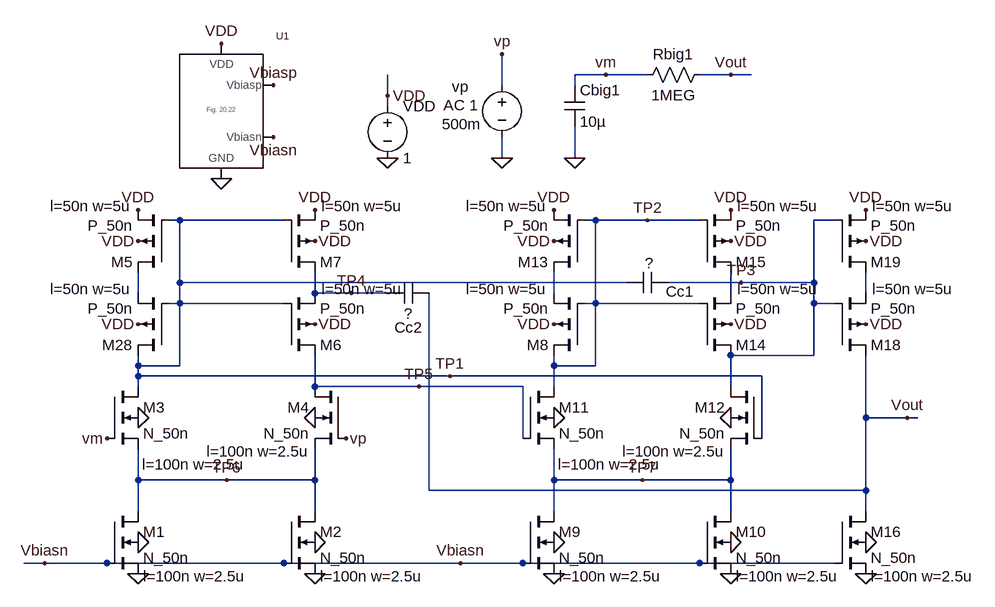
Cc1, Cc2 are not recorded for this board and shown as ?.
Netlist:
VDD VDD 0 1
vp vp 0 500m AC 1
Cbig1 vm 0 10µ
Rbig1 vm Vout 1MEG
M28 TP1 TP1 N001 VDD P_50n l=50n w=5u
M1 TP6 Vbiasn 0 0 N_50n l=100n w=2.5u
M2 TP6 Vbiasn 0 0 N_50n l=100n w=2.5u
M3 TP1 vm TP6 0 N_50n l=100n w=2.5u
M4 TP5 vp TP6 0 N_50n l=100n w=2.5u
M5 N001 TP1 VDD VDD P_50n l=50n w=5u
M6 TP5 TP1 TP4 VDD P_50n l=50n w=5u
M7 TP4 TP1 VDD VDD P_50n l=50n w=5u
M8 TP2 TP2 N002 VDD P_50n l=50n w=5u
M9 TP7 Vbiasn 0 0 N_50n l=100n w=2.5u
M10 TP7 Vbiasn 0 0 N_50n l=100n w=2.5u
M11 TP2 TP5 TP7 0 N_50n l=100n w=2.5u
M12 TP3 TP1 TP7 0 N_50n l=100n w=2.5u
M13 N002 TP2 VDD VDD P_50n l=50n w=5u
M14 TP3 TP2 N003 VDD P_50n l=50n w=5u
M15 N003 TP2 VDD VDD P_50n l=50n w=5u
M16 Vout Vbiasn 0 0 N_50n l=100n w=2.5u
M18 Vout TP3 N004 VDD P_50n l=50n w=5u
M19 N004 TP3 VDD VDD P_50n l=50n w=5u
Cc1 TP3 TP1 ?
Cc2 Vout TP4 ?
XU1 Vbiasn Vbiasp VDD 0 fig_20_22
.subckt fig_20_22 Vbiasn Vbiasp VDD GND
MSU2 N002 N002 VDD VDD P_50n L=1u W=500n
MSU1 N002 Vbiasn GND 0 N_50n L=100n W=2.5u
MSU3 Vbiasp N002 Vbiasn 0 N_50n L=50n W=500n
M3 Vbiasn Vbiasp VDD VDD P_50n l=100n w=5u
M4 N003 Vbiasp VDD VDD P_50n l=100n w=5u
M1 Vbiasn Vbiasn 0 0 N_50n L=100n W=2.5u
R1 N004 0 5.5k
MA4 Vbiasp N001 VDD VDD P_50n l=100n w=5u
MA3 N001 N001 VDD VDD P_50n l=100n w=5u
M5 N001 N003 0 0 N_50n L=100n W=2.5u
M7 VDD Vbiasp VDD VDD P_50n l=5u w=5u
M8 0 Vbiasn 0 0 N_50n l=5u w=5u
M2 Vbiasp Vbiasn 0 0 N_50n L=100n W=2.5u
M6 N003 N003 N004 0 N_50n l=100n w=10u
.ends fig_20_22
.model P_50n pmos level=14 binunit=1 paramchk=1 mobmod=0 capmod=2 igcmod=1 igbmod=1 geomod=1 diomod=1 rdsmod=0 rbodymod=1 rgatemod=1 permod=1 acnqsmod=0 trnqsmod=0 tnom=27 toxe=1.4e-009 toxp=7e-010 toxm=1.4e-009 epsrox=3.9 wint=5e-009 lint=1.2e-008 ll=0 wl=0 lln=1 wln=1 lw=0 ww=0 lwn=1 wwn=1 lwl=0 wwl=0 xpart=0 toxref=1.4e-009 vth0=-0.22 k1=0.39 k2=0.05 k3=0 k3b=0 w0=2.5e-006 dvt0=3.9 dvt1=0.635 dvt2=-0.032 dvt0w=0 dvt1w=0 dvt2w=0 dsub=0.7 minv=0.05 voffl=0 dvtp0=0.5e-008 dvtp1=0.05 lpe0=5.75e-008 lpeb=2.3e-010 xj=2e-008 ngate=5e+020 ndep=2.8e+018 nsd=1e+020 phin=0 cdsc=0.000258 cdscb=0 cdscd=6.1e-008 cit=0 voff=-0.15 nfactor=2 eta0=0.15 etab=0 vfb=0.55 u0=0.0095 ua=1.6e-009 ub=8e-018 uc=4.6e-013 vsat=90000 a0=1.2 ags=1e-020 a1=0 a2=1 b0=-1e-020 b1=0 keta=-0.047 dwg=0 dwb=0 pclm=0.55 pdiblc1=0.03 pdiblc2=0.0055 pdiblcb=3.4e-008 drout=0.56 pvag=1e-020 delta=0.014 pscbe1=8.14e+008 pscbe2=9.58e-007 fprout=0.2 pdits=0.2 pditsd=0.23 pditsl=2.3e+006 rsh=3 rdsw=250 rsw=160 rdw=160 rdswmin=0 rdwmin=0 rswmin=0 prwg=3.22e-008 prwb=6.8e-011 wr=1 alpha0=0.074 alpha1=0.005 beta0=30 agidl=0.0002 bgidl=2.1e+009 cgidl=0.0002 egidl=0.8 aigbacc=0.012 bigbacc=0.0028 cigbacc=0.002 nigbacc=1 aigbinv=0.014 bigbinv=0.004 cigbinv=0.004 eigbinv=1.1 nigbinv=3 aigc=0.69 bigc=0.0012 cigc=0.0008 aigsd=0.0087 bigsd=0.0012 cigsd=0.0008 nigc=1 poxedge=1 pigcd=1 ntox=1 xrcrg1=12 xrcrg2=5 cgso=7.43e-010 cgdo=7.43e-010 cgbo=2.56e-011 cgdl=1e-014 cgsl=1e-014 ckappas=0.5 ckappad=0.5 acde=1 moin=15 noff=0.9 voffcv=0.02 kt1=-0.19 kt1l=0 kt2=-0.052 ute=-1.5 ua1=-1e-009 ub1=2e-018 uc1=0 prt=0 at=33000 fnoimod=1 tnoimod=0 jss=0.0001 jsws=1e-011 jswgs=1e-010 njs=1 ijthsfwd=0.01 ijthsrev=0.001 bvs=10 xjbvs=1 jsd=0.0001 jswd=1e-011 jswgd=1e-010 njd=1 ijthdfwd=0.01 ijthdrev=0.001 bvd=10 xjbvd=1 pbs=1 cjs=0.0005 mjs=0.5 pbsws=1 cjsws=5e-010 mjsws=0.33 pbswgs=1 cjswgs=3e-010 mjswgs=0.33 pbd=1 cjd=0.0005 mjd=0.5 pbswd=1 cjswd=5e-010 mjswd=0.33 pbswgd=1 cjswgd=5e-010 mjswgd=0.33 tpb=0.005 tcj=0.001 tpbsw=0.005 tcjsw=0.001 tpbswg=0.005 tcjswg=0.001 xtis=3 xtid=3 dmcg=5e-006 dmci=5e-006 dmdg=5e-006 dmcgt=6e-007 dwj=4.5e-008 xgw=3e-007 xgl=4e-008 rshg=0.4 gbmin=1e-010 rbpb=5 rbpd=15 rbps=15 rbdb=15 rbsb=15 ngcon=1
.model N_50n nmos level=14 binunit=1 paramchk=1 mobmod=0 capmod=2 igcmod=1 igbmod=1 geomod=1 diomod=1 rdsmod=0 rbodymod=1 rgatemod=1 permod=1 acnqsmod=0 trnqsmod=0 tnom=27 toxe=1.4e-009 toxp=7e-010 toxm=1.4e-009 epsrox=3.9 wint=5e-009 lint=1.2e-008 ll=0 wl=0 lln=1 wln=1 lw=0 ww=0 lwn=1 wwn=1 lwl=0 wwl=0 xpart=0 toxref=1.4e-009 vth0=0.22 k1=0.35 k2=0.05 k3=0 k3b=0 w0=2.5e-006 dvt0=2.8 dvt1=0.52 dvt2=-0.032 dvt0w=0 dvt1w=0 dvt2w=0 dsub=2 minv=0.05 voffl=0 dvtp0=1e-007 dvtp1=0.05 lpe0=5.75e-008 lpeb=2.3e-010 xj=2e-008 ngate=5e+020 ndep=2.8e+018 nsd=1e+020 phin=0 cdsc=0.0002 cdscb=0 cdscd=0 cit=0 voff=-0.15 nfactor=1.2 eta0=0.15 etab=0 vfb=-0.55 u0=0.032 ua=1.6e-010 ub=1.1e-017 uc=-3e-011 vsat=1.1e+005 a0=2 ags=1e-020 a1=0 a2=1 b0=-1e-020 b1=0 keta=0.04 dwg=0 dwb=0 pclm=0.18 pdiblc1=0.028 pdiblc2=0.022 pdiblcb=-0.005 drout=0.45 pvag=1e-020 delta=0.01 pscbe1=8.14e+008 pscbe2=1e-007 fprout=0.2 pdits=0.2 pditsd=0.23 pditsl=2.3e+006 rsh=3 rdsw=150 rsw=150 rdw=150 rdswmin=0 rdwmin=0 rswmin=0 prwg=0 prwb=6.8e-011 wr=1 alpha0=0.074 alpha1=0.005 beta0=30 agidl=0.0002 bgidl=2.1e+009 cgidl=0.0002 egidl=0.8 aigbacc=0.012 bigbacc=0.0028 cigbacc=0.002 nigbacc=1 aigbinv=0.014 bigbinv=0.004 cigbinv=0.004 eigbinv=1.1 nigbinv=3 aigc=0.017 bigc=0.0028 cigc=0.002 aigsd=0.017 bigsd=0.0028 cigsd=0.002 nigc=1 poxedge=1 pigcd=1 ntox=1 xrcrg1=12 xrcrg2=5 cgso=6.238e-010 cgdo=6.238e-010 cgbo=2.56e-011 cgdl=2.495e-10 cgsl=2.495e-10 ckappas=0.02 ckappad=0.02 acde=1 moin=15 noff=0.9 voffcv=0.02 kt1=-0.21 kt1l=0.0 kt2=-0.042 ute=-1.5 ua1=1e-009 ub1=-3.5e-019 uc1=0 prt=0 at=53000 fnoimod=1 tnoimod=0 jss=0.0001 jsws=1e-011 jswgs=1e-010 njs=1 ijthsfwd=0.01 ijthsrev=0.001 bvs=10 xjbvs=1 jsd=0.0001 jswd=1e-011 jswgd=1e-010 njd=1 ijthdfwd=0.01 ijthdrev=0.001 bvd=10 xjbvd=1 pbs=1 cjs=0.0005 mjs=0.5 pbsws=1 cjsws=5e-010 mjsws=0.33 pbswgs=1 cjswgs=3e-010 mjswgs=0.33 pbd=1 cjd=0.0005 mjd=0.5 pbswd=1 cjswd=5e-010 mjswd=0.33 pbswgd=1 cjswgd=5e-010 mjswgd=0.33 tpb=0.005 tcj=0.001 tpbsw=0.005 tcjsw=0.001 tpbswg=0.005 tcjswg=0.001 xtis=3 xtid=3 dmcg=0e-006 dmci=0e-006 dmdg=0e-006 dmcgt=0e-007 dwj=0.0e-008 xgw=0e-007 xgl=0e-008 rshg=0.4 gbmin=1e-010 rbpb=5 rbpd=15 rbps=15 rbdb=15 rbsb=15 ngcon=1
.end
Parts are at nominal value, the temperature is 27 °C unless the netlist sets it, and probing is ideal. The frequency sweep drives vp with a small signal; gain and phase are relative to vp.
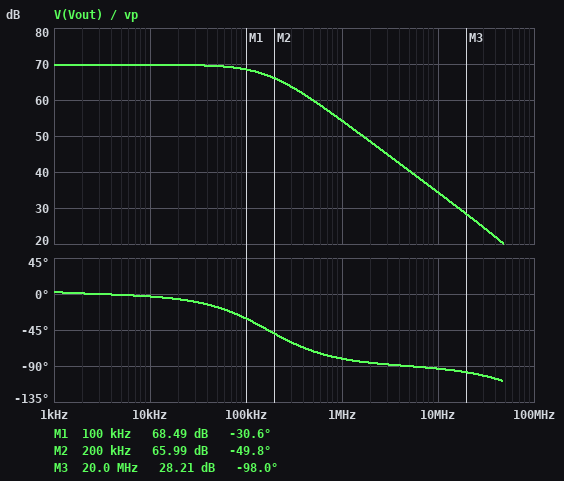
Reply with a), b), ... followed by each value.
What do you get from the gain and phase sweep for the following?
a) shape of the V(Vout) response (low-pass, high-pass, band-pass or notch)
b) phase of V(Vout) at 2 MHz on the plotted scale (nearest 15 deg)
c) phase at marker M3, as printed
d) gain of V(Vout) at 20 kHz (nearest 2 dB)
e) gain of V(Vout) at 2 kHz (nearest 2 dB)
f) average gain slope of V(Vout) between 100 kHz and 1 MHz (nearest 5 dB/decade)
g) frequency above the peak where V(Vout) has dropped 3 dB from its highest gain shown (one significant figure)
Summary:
a) low-pass
b) -90 deg
c) -98.0 deg
d) 70 dB
e) 70 dB
f) -15 dB/decade
g) 200 kHz
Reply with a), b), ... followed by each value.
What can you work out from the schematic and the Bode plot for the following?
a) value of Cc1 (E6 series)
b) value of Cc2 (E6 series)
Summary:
a) 100 fF
b) 68 fF
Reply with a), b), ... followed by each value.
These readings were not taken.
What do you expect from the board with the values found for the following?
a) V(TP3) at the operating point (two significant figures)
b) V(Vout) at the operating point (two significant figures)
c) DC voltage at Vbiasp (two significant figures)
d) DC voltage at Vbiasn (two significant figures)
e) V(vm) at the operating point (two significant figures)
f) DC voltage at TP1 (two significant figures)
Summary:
a) 670 mV
b) 500 mV
c) 650 mV
d) 350 mV
e) 500 mV
f) 680 mV
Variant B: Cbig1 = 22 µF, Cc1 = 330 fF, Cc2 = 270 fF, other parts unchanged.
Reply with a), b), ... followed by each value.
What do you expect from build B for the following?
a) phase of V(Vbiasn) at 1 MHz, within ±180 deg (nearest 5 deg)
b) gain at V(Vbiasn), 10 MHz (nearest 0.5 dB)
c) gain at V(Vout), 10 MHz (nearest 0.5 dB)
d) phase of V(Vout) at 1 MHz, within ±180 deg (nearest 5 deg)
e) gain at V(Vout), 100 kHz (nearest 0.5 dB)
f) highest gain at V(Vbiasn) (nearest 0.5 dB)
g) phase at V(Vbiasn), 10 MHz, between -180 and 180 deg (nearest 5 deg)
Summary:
a) 0 deg
b) -36.0 dB
c) 22.5 dB
d) -90 deg
e) 62.0 dB
f) -34.5 dB
g) -40 deg
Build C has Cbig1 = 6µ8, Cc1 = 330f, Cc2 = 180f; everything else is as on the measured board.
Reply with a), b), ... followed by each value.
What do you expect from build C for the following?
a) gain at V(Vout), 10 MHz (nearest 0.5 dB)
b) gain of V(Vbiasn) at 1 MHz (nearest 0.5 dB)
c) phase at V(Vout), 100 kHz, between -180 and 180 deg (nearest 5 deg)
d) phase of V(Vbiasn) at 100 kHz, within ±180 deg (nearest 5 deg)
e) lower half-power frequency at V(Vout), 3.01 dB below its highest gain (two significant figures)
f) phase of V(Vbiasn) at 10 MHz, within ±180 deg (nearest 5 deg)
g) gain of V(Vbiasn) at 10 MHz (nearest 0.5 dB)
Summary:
a) 25.5 dB
b) -31.5 dB
c) -60 deg
d) 25 deg
e) 72 Hz
f) -40 deg
g) -33.5 dB
